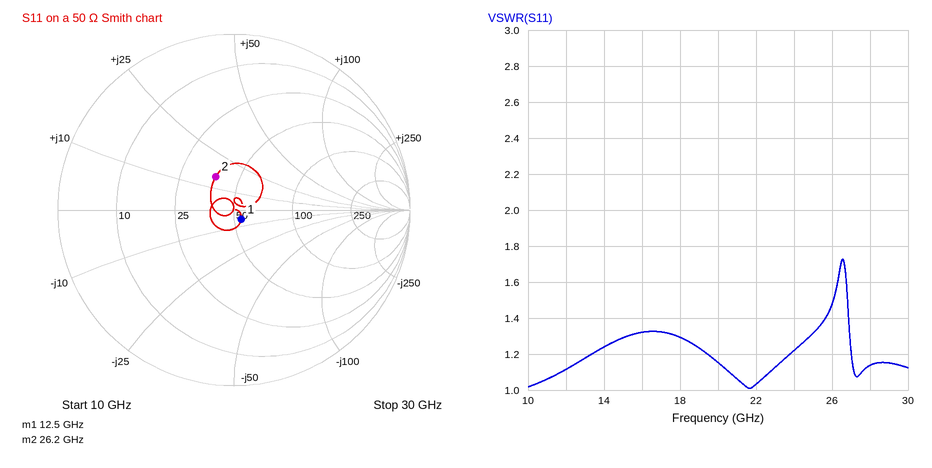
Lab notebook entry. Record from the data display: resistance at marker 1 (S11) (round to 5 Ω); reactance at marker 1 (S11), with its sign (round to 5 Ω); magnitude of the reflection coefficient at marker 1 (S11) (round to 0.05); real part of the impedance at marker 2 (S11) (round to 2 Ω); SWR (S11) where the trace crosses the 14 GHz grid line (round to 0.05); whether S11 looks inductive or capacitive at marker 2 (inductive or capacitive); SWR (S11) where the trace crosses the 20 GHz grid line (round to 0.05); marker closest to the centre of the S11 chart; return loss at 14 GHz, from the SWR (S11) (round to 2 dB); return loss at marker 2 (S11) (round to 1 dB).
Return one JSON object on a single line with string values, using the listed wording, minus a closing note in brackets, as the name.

{"resistance at marker 1 (S11)": "55 Ω", "reactance at marker 1 (S11), with its sign": "-5 Ω", "magnitude of the reflection coefficient at marker 1 (S11)": "0.05", "real part of the impedance at marker 2 (S11)": "38 Ω", "SWR (S11) where the trace crosses the 14 GHz grid line": "1.25", "whether S11 looks inductive or capacitive at marker 2": "inductive", "SWR (S11) where the trace crosses the 20 GHz grid line": "1.15", "marker closest to the centre of the S11 chart": "marker 1", "return loss at 14 GHz, from the SWR (S11)": "20 dB", "return loss at marker 2 (S11)": "13 dB"}
